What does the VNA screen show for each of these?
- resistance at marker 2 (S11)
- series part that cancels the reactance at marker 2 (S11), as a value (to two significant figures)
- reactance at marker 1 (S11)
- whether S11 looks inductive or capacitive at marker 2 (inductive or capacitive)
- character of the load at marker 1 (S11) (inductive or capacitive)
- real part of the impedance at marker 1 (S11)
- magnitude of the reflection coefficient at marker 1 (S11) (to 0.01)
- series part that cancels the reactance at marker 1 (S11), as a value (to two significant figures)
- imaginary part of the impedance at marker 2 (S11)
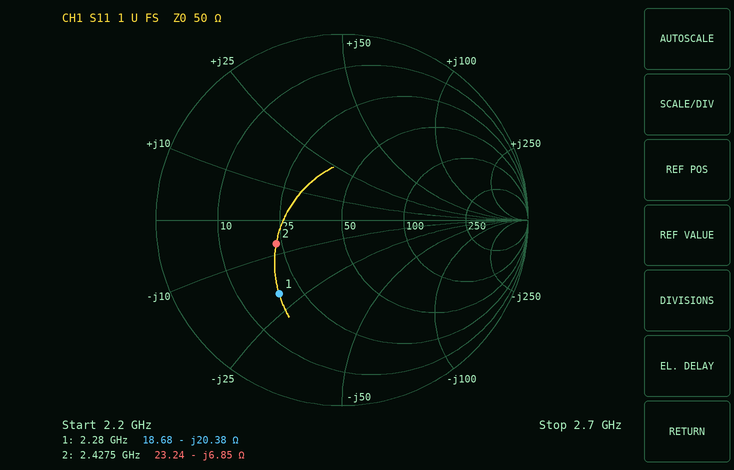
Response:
23.24 Ω
450 pH
-20.38 Ω
capacitive
capacitive
18.68 Ω
0.52
1.4 nH
-6.85 Ω
